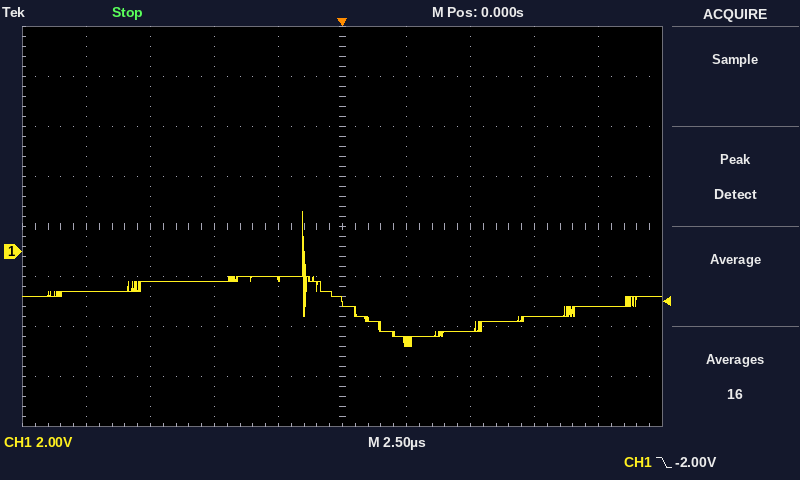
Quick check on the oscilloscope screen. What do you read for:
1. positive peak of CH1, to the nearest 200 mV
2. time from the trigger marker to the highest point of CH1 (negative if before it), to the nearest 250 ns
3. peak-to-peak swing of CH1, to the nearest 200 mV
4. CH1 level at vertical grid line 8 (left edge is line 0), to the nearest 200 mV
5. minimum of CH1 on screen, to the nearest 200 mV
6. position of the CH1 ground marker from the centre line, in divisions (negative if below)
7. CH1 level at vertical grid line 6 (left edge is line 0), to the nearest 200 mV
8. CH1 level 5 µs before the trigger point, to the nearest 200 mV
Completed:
1.6 V
-1.50 µs
5.4 V
-2.6 V
-3.8 V
-0.5 div
-3.6 V
-1.2 V
